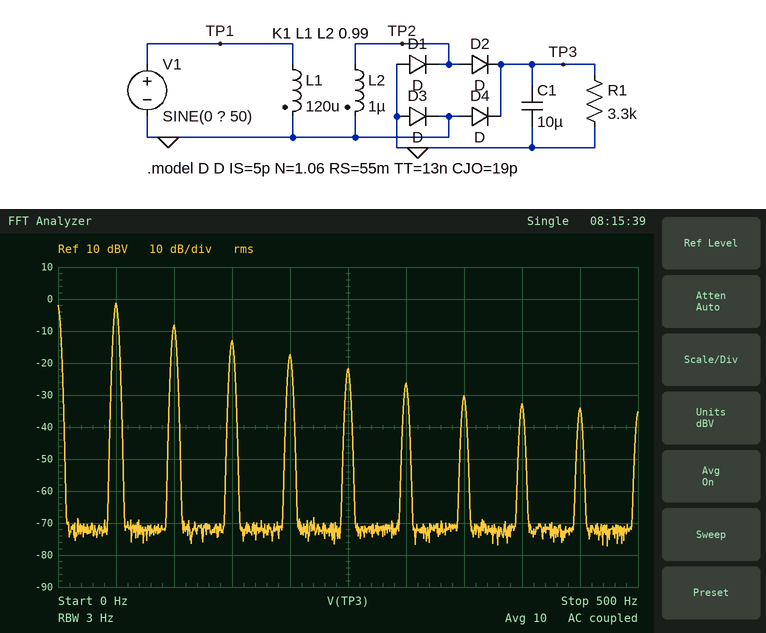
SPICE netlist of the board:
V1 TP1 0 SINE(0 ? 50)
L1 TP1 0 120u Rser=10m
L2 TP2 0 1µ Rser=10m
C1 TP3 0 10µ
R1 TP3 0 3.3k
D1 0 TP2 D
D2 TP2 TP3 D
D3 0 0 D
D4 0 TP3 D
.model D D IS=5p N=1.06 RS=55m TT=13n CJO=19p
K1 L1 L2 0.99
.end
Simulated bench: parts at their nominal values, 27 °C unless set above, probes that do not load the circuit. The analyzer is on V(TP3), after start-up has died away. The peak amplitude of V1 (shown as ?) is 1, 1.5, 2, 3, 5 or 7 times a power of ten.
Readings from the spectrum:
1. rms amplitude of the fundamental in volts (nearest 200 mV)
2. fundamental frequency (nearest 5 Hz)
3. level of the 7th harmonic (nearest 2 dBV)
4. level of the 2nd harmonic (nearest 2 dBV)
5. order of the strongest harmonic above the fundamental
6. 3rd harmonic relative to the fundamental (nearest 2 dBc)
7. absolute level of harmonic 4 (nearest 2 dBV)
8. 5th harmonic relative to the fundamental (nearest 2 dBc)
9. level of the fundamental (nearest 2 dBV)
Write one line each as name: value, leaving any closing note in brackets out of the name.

rms amplitude of the fundamental in volts: 800 mV
fundamental frequency: 50 Hz
level of the 7th harmonic: -30 dBV
level of the 2nd harmonic: -8 dBV
order of the strongest harmonic above the fundamental: 2
3rd harmonic relative to the fundamental: -12 dBc
absolute level of harmonic 4: -18 dBV
5th harmonic relative to the fundamental: -20 dBc
level of the fundamental: -2 dBV
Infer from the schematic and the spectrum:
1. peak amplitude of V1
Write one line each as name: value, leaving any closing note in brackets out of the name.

peak amplitude of V1: 100 V
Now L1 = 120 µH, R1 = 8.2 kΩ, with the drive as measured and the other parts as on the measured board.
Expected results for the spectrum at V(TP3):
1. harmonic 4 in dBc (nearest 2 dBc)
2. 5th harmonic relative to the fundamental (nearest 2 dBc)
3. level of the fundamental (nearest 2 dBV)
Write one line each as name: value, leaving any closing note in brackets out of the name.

harmonic 4 in dBc: -14 dBc
5th harmonic relative to the fundamental: -16 dBc
level of the fundamental: -8 dBV
